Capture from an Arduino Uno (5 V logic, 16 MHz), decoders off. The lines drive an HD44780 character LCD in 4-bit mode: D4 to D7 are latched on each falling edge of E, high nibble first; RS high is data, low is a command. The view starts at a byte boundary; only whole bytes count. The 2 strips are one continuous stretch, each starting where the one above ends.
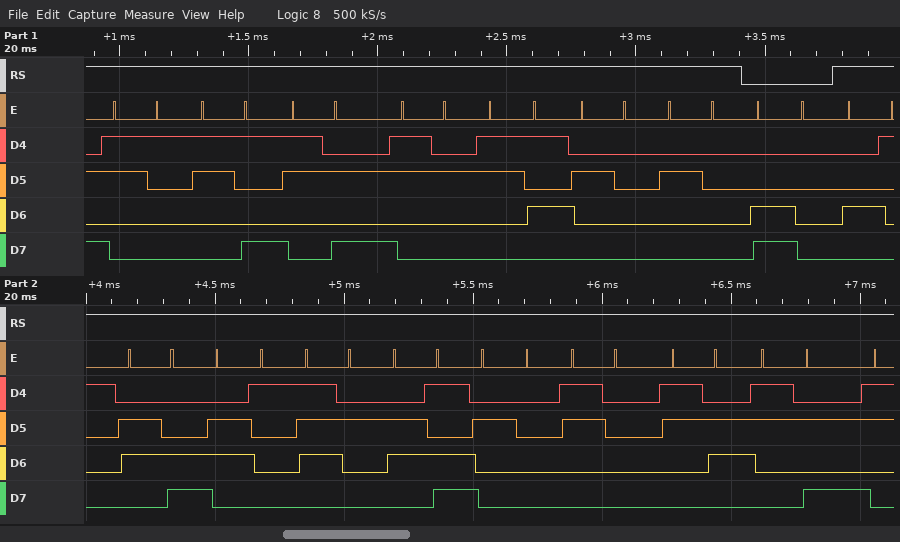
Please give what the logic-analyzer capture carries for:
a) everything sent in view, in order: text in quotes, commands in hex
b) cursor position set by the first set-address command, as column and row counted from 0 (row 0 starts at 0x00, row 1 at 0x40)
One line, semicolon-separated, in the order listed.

"19:25  " 0xC0 "Alarm 06:"; column 0, row 1
